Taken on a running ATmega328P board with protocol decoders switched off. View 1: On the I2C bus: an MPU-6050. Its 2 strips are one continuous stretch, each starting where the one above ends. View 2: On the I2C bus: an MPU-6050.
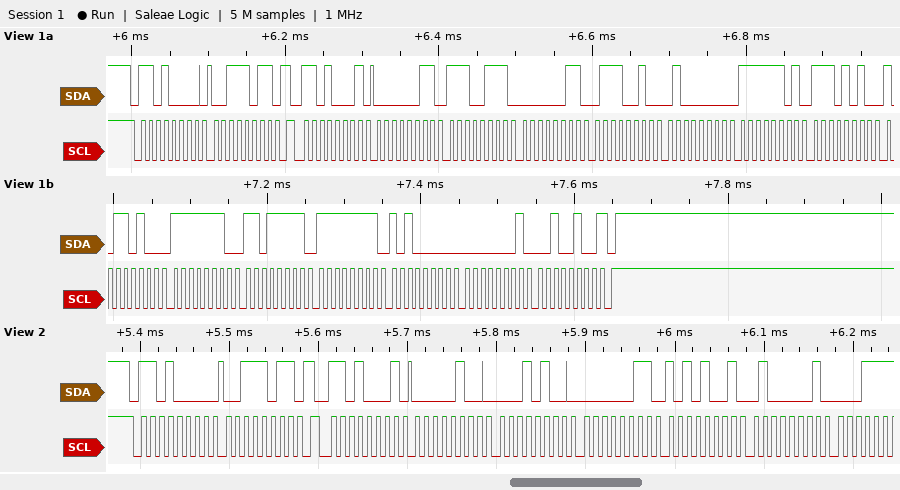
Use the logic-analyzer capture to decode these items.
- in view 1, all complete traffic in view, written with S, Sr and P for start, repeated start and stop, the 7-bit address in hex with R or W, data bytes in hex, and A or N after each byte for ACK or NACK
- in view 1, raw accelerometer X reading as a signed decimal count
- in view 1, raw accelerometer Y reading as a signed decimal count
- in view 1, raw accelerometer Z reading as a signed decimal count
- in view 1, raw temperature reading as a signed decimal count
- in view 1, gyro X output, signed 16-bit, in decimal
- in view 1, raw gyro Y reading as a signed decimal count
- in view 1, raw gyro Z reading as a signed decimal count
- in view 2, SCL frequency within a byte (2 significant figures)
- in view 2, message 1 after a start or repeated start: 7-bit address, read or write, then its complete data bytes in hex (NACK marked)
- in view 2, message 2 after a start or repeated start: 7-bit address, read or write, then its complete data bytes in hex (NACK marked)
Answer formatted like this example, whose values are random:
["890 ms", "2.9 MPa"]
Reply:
["S 68W A 3B A Sr 68R A 03 A E7 A 03 A 72 A 40 A FD A EA A B4 A FE A DF A FF A A0 A 01 A 24 N P", "999", "882", "16637", "-5452", "-289", "-96", "292", "100 kHz", "0x68 write: 3B", "0x68 read: 04 14 03 A9 41"]
